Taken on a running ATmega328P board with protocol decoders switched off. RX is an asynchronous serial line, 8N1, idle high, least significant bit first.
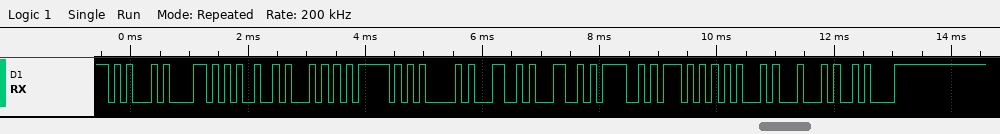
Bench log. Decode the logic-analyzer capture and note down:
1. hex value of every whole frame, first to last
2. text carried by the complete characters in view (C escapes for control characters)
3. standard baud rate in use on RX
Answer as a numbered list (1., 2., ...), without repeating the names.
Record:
1. 0x45 0x58 0x49 0x54 0x5F 0x41 0x4C 0x4C 0x4F 0x57 0x45 0x44 0x0A
2. "EXIT_ALLOWED\n"
3. 9600 baud
